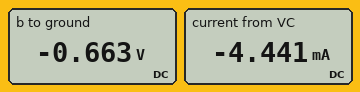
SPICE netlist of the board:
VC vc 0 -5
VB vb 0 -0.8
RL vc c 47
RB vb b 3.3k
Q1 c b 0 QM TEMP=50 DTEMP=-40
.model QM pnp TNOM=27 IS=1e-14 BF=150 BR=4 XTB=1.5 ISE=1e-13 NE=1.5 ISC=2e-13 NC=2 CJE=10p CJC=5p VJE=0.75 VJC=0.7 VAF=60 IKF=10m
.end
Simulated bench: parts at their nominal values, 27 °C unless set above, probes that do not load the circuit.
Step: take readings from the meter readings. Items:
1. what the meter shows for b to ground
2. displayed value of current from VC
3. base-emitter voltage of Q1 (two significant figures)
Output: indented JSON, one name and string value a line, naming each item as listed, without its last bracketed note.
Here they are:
{
  "what the meter shows for b to ground": "-0.663 V",
  "displayed value of current from VC": "-4.441 mA",
  "base-emitter voltage of Q1": "-660 mV"
}
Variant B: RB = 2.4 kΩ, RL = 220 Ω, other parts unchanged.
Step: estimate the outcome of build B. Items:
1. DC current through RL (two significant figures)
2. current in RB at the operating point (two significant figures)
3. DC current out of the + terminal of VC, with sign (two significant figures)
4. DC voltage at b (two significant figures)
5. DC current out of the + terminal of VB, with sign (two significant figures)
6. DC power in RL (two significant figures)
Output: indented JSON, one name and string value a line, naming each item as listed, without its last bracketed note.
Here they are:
{
  "DC current through RL": "5.4 mA",
  "current in RB at the operating point": "54 µA",
  "DC current out of the + terminal of VC, with sign": "-5.4 mA",
  "DC voltage at b": "-670 mV",
  "DC current out of the + terminal of VB, with sign": "-54 µA",
  "DC power in RL": "6.4 mW"
}
